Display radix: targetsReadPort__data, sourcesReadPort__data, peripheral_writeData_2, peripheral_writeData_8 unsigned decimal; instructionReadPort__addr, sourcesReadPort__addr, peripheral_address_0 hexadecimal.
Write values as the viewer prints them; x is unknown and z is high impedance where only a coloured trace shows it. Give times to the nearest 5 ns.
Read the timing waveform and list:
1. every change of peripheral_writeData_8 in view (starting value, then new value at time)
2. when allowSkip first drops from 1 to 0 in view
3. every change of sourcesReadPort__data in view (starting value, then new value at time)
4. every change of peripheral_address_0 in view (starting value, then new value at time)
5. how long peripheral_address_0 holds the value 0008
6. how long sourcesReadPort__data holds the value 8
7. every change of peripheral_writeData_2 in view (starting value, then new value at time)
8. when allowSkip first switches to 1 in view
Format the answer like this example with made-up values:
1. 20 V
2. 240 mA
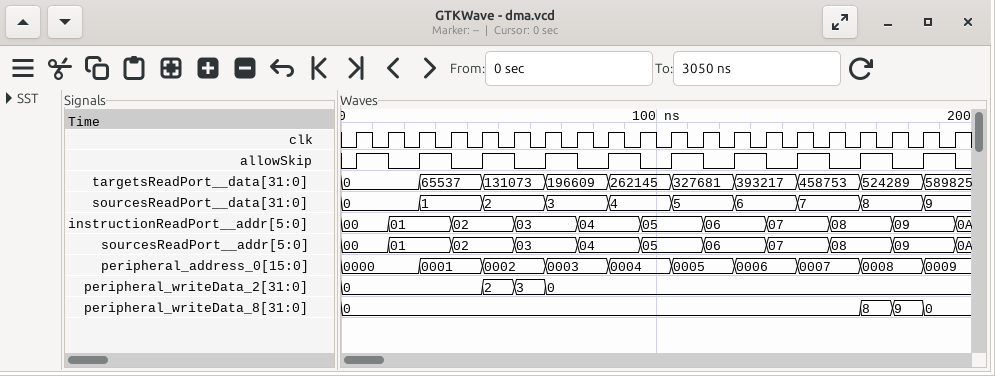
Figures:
1. 0, 8 at 165 ns, 9 at 175 ns, 0 at 185 ns
2. 15 ns
3. 0, 1 at 25 ns, 2 at 45 ns, 3 at 65 ns, 4 at 85 ns, 5 at 105 ns, 6 at 125 ns, 7 at 145 ns, 8 at 165 ns, 9 at 185 ns
4. 0000, 0001 at 25 ns, 0002 at 45 ns, 0003 at 65 ns, 0004 at 85 ns, 0005 at 105 ns, 0006 at 125 ns, 0007 at 145 ns, 0008 at 165 ns, 0009 at 185 ns
5. 20 ns
6. 20 ns
7. 0, 2 at 45 ns, 3 at 55 ns, 0 at 65 ns
8. 5 ns
